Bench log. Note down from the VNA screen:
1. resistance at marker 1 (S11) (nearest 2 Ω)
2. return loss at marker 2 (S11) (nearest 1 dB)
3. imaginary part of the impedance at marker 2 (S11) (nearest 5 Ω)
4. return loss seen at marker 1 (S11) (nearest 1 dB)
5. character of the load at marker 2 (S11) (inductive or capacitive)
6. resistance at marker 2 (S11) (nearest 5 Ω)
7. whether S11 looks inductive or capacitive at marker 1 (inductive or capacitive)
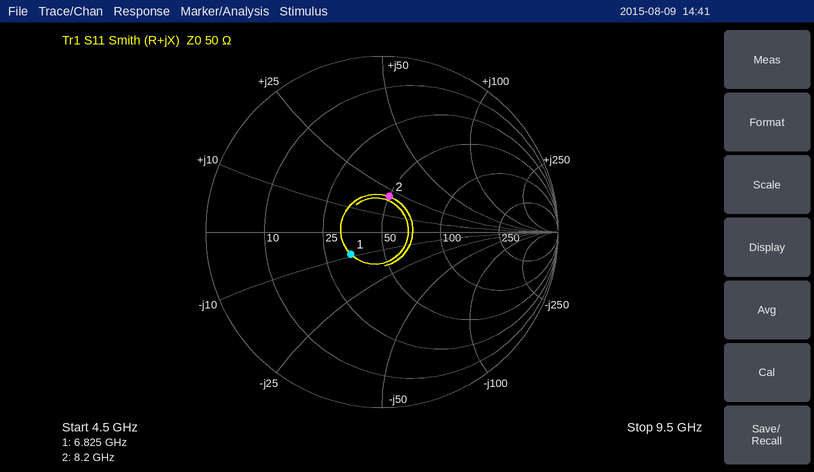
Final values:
34 Ω
14 dB
+20 Ω
13 dB
inductive
50 Ω
capacitive
